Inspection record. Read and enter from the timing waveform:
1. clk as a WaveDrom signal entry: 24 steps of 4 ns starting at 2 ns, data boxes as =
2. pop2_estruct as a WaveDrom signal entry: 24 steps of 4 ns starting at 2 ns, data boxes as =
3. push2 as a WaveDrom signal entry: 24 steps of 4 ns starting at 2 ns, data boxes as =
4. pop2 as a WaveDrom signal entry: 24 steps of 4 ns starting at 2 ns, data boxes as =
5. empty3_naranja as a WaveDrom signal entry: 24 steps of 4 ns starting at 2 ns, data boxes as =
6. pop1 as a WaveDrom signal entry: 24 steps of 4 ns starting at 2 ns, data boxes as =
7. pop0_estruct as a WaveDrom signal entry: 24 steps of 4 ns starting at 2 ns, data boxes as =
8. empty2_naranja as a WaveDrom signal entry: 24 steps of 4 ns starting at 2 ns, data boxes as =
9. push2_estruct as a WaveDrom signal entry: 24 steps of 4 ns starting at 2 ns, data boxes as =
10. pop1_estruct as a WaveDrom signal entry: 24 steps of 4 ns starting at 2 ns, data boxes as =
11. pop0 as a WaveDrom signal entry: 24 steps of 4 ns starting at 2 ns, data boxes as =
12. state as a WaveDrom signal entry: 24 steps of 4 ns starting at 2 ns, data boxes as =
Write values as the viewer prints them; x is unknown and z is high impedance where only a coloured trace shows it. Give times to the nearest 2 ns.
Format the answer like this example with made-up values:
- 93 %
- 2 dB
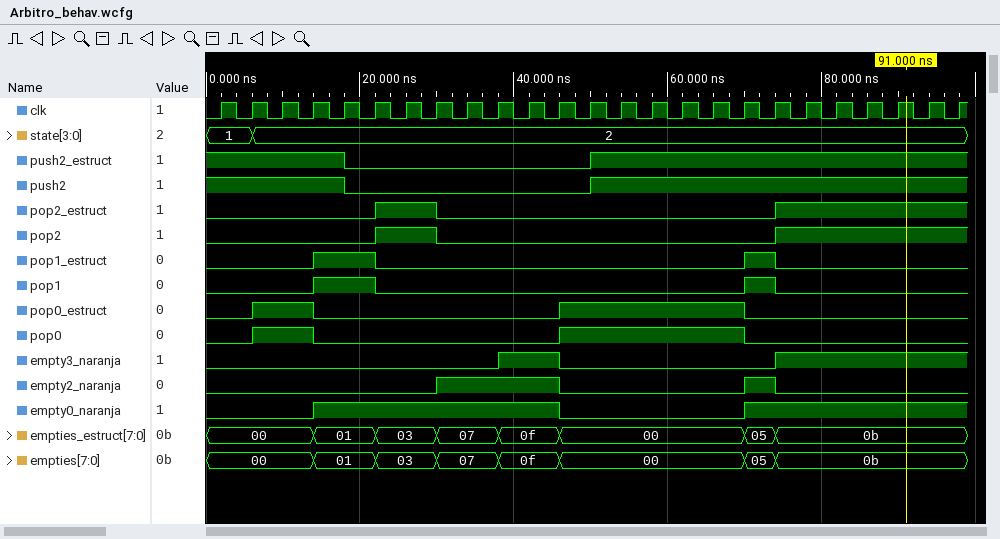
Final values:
- {name: 'clk', wave: 'p.......................'}
- {name: 'pop2_estruct', wave: '0....1.0..........1.....'}
- {name: 'push2', wave: '1...0.......1...........'}
- {name: 'pop2', wave: '0....1.0..........1.....'}
- {name: 'empty3_naranja', wave: '0........1.0......1.....'}
- {name: 'pop1', wave: '0..1.0...........10.....'}
- {name: 'pop0_estruct', wave: '01.0.......1.....0......'}
- {name: 'empty2_naranja', wave: '0......1...0.....10.....'}
- {name: 'push2_estruct', wave: '1...0.......1...........'}
- {name: 'pop1_estruct', wave: '0..1.0...........10.....'}
- {name: 'pop0', wave: '01.0.......1.....0......'}
- {name: 'state', wave: '==......................', data: '1 2'}
